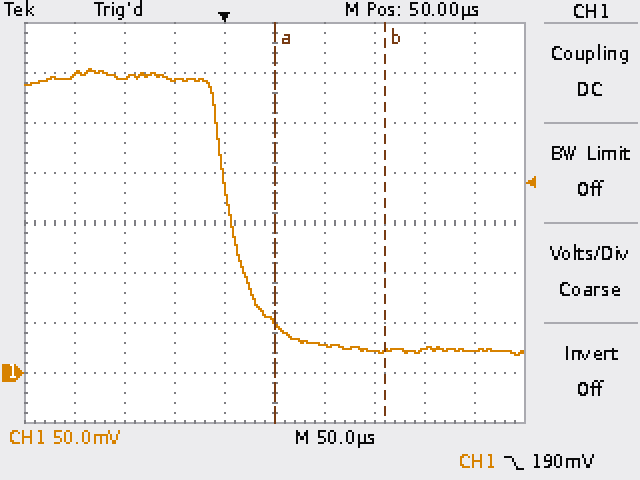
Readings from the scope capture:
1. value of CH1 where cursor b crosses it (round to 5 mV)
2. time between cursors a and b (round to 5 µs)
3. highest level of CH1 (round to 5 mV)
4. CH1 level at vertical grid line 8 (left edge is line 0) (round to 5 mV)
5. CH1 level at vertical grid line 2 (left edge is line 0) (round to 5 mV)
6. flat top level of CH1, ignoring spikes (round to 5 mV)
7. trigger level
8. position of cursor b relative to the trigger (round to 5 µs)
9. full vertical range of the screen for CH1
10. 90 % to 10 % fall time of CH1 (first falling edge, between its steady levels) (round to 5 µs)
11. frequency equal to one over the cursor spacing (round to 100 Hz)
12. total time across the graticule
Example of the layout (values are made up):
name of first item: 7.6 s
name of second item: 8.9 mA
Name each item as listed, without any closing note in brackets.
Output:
value of CH1 where cursor b crosses it: 20 mV
time between cursors a and b: 110 µs
highest level of CH1: 305 mV
CH1 level at vertical grid line 8 (left edge is line 0): 25 mV
CH1 level at vertical grid line 2 (left edge is line 0): 295 mV
flat top level of CH1, ignoring spikes: 295 mV
trigger level: 190 mV
position of cursor b relative to the trigger: +160 µs
full vertical range of the screen for CH1: 400 mV
90 % to 10 % fall time of CH1 (first falling edge, between its steady levels): 60 µs
frequency equal to one over the cursor spacing: 9.1 kHz
total time across the graticule: 500 µs
